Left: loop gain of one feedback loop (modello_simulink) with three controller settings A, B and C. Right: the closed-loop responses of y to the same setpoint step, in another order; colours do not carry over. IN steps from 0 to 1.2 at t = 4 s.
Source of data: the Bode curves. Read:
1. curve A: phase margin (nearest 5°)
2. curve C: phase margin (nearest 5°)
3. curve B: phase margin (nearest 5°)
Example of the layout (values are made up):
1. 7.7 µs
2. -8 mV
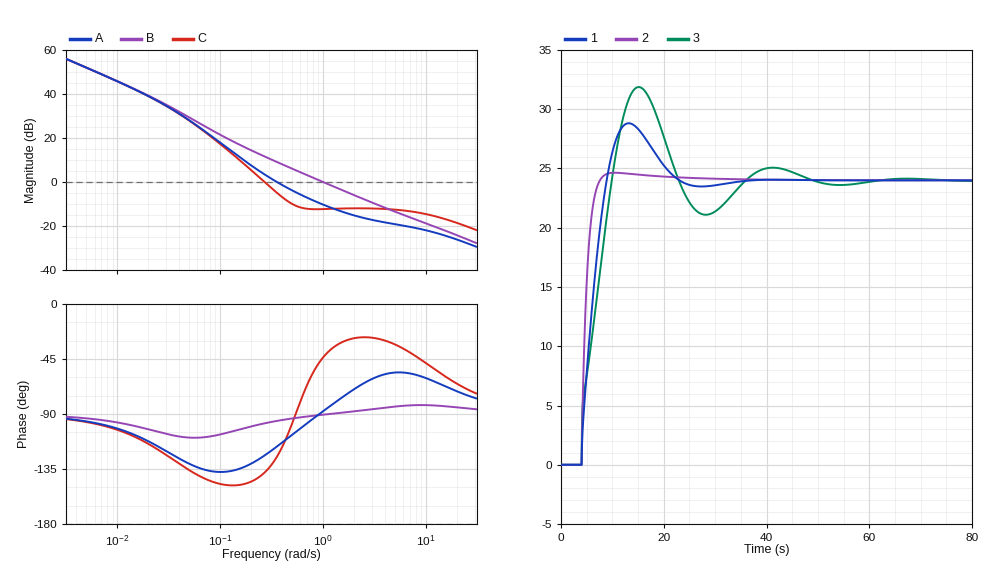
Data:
1. 65°
2. 40°
3. 90°
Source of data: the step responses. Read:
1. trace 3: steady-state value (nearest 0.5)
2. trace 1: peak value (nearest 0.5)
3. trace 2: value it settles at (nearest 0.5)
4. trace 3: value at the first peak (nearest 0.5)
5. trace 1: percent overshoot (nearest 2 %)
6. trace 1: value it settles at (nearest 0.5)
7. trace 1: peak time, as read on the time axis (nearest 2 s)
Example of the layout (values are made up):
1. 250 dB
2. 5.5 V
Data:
1. 24.0
2. 29.0
3. 24.0
4. 32.0
5. 20 %
6. 24.0
7. 14 s
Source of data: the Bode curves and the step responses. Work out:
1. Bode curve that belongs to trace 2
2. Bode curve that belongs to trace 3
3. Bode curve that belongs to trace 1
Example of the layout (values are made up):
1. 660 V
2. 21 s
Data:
1. B
2. C
3. A
